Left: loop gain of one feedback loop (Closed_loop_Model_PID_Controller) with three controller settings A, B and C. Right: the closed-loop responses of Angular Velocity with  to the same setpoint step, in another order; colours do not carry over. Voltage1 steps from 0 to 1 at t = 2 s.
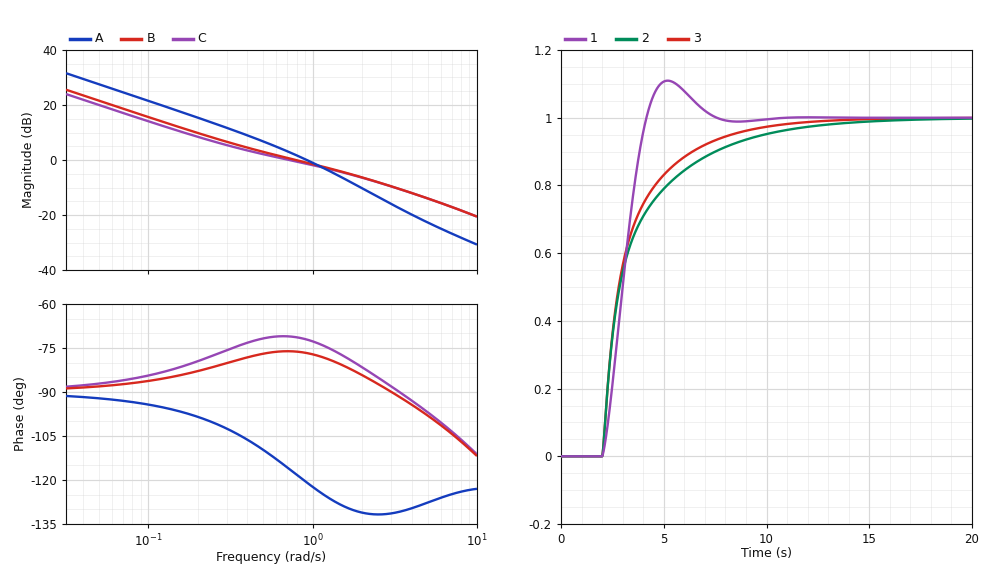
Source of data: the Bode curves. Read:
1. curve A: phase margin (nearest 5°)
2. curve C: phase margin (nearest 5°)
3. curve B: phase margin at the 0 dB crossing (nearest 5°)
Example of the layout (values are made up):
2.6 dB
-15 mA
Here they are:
60°
110°
105°
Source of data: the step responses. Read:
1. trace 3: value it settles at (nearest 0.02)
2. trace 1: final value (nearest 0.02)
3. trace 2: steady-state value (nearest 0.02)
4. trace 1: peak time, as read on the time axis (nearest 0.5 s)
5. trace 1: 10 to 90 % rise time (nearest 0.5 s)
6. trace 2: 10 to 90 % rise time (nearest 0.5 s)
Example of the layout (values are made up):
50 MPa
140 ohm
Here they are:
1.00
1.00
1.00
5.0 s
1.5 s
5.5 s
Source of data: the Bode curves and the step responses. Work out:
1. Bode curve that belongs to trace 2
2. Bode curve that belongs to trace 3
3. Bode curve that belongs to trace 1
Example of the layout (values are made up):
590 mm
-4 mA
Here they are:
C
B
A
